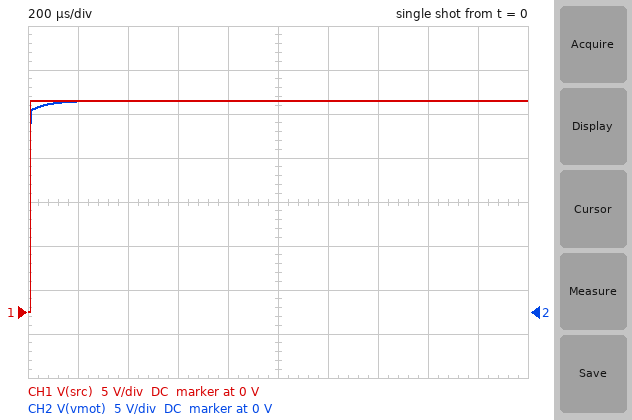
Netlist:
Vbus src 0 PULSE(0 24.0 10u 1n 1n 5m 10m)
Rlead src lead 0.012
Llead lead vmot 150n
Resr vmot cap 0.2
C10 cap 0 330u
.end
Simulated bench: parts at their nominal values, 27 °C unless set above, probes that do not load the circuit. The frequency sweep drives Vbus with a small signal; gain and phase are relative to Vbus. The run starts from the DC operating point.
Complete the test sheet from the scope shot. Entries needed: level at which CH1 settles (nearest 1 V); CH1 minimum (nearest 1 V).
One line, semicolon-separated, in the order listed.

24 V; 0 V
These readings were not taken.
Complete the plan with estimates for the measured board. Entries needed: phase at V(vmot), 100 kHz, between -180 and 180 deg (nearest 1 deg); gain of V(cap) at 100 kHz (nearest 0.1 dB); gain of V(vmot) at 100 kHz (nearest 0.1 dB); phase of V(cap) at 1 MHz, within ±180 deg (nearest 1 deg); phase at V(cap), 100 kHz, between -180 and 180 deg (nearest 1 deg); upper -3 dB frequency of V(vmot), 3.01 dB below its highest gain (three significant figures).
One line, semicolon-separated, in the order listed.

-24 deg; -33.6 dB; -1.2 dB; -167 deg; -113 deg; 201 kHz
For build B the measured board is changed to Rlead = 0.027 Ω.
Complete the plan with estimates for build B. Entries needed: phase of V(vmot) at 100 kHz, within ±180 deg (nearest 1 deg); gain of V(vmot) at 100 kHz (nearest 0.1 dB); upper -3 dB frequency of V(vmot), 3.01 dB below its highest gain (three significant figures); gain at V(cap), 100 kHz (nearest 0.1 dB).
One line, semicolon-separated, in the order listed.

-23 deg; -1.7 dB; 182 kHz; -34.1 dB
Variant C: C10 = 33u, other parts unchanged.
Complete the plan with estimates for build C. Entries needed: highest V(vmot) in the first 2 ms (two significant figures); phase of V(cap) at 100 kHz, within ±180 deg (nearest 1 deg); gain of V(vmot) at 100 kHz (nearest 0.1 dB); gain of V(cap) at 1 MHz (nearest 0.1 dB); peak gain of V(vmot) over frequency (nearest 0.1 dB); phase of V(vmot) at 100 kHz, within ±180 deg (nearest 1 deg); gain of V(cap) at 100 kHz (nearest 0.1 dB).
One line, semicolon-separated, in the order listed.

25 V; -102 deg; -0.5 dB; -46.0 dB; 0.2 dB; -26 deg; -13.1 dB
